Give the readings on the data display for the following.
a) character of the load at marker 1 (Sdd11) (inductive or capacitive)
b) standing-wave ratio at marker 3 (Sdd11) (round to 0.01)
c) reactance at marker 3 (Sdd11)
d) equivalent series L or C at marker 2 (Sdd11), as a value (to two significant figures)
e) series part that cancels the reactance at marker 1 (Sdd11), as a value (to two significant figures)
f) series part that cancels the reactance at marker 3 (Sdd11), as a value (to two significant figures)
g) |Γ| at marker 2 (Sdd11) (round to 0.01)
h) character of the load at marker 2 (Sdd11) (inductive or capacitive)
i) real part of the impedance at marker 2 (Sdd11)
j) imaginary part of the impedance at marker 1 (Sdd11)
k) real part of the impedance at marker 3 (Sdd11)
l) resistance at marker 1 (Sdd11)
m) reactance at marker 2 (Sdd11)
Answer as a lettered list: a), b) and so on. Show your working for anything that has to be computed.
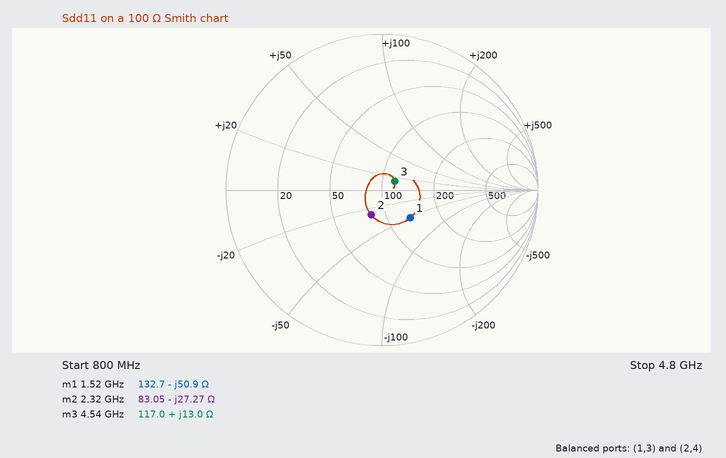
a) capacitive
b) 1.22
c) +13.0 Ω
d) C = 1/(2π × 2.32 GHz × 27.27 Ω) ≈ 2.5 pF
e) L = 50.9 Ω/(2π × 1.52 GHz) ≈ 5.3 nH
f) C = 1/(2π × 4.54 GHz × 13 Ω) ≈ 2.7 pF
g) 0.17
h) capacitive
i) 83.05 Ω
j) -50.9 Ω
k) 117.0 Ω
l) 132.7 Ω
m) -27.27 Ω
